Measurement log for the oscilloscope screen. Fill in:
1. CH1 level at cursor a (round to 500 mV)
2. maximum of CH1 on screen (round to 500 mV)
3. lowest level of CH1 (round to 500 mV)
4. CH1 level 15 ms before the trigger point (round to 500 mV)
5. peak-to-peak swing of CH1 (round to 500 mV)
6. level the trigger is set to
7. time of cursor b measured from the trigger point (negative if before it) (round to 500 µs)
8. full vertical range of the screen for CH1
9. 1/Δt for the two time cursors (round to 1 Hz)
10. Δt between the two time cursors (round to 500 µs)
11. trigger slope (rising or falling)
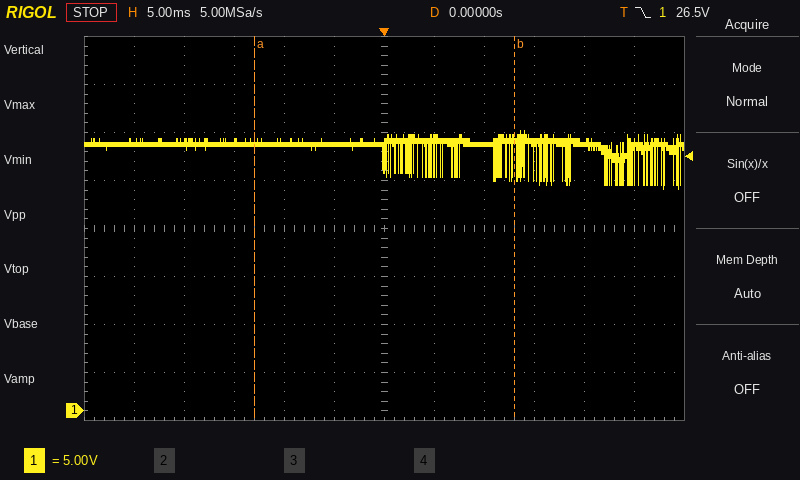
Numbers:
28.0 V
29.0 V
23.0 V
28.0 V
6.0 V
26.5 V
+13.0 ms
40 V
38 Hz
26.0 ms
falling
